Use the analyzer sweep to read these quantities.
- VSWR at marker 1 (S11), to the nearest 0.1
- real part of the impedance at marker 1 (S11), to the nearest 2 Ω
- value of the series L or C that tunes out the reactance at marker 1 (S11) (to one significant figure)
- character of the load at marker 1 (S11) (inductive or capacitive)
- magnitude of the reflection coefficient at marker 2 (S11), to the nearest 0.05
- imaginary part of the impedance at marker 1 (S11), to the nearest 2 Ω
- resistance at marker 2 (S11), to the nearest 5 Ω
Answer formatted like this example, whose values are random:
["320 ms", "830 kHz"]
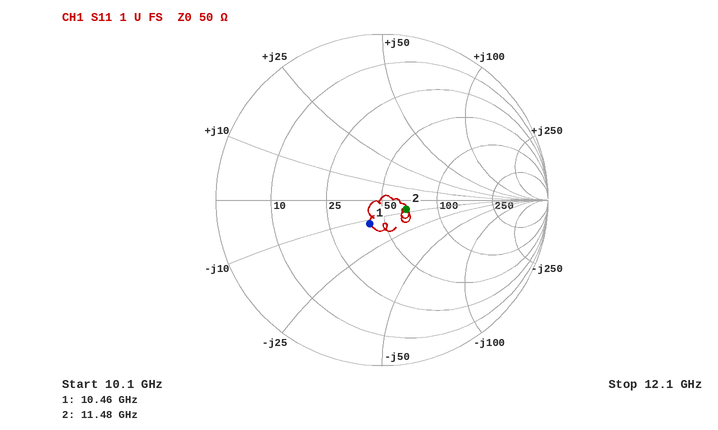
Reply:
["1.4", "42 Ω", "200 pH", "capacitive", "0.15", "-12 Ω", "65 Ω"]
